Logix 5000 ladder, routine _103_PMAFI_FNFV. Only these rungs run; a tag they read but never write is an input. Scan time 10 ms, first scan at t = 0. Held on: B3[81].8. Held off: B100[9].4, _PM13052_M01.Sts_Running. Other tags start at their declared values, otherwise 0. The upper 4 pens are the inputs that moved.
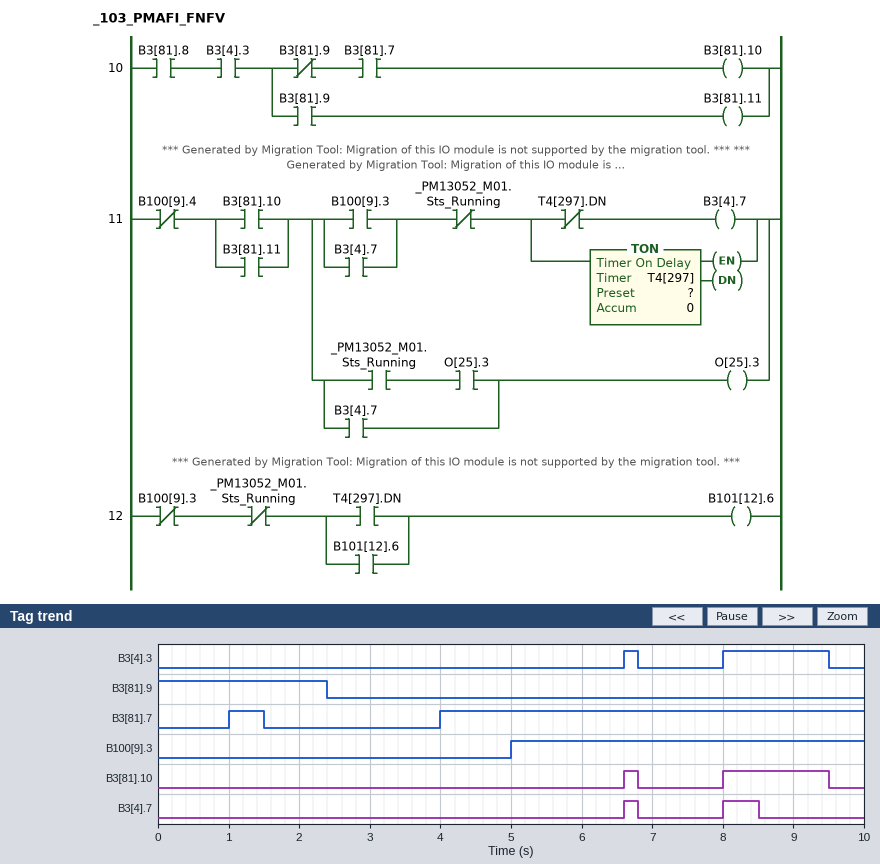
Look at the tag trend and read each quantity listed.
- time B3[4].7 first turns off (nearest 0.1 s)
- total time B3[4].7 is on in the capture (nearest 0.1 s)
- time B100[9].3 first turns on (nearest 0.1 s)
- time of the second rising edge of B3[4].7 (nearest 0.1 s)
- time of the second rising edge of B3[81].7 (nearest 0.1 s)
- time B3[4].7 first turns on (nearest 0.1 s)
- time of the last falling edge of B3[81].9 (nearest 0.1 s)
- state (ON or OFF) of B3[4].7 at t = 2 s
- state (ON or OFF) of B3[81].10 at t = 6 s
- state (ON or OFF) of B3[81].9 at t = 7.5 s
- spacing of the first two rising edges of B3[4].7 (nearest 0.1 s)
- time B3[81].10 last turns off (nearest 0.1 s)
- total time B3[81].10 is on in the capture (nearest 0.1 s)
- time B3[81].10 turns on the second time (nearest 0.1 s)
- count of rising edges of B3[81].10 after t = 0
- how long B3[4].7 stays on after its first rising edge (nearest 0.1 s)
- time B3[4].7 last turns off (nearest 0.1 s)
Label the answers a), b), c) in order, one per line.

a) 6.8 s
b) 0.7 s
c) 5.0 s
d) 8.0 s
e) 4.0 s
f) 6.6 s
g) 2.4 s
h) OFF
i) OFF
j) OFF
k) 1.4 s
l) 9.5 s
m) 1.7 s
n) 8.0 s
o) 2
p) 0.2 s
q) 8.5 s
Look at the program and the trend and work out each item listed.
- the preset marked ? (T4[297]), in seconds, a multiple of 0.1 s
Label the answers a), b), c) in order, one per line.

a) 0.5 s
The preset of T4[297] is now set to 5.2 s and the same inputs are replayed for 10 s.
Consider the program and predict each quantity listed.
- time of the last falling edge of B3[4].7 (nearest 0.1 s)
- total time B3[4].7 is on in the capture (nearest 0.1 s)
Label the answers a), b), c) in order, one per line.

a) 9.5 s
b) 1.7 s
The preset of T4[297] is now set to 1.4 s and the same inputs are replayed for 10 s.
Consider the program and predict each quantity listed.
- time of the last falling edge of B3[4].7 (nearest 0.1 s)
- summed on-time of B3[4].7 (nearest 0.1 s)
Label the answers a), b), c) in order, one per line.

a) 9.4 s
b) 1.6 s
